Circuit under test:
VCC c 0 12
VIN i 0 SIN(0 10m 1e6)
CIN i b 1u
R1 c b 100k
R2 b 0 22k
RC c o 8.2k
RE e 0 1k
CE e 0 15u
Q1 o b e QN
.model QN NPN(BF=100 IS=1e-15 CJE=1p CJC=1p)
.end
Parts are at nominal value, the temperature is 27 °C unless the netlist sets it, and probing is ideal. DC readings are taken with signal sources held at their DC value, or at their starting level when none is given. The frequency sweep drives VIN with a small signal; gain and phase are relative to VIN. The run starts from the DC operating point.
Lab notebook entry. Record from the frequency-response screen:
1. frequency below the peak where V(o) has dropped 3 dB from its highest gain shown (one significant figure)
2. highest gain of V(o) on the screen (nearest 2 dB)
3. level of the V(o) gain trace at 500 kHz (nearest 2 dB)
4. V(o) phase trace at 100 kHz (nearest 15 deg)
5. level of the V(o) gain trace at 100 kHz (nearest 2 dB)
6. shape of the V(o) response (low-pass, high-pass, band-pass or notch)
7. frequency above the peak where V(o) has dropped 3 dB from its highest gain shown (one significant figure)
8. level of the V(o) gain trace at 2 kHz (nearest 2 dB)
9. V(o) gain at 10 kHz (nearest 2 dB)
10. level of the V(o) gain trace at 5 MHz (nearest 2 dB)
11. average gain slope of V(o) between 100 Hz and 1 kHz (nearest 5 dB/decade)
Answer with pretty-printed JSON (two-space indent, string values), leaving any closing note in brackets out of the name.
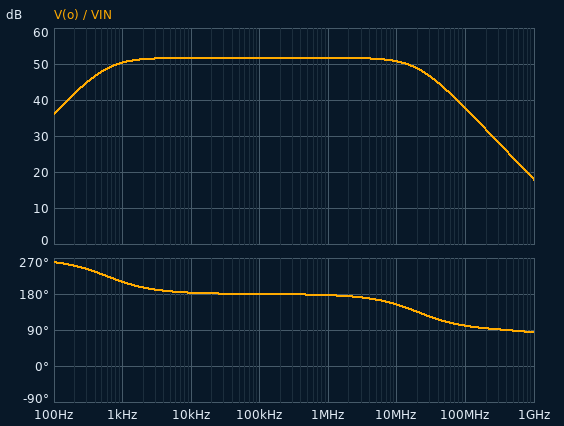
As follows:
{
  "frequency below the peak where V(o) has dropped 3 dB from its highest gain shown": "600 Hz",
  "highest gain of V(o) on the screen": "52 dB",
  "level of the V(o) gain trace at 500 kHz": "52 dB",
  "V(o) phase trace at 100 kHz": "180 deg",
  "level of the V(o) gain trace at 100 kHz": "52 dB",
  "shape of the V(o) response": "band-pass",
  "frequency above the peak where V(o) has dropped 3 dB from its highest gain shown": "20 MHz",
  "level of the V(o) gain trace at 2 kHz": "52 dB",
  "V(o) gain at 10 kHz": "52 dB",
  "level of the V(o) gain trace at 5 MHz": "52 dB",
  "average gain slope of V(o) between 100 Hz and 1 kHz": "15 dB/decade"
}
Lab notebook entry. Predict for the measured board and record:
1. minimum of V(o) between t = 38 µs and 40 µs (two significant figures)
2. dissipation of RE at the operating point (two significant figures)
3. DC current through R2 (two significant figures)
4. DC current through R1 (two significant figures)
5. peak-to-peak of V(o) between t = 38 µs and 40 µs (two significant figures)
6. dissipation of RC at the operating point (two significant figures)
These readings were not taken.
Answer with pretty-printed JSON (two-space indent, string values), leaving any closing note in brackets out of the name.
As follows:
{
  "minimum of V(o) between t = 38 µs and 40 µs": "1.3 V",
  "dissipation of RE at the operating point": "1.5 mW",
  "DC current through R2": "88 µA",
  "DC current through R1": "100 µA",
  "peak-to-peak of V(o) between t = 38 µs and 40 µs": "4.4 V",
  "dissipation of RC at the operating point": "12 mW"
}
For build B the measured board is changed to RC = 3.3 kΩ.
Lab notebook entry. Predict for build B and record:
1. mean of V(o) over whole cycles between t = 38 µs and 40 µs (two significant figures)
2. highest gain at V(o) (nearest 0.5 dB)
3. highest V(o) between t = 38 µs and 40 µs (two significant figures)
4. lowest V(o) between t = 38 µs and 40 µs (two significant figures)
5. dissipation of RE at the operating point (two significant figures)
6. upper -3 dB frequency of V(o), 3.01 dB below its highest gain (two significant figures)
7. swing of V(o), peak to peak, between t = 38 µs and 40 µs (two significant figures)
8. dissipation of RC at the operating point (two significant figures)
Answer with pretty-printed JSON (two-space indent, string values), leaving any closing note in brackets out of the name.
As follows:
{
  "mean of V(o) over whole cycles between t = 38 µs and 40 µs": "7.9 V",
  "highest gain at V(o)": "44.0 dB",
  "highest V(o) between t = 38 µs and 40 µs": "9.3 V",
  "lowest V(o) between t = 38 µs and 40 µs": "6.1 V",
  "dissipation of RE at the operating point": "1.5 mW",
  "upper -3 dB frequency of V(o), 3.01 dB below its highest gain": "100 MHz",
  "swing of V(o), peak to peak, between t = 38 µs and 40 µs": "3.2 V",
  "dissipation of RC at the operating point": "4.9 mW"
}
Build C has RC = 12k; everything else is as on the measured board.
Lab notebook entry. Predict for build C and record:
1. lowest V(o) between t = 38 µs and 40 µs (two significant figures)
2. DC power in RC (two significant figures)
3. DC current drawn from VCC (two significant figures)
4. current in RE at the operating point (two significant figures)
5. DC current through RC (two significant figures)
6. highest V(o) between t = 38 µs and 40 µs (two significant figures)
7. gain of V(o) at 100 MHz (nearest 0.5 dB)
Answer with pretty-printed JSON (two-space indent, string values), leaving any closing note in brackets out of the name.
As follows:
{
  "lowest V(o) between t = 38 µs and 40 µs": "990 mV",
  "DC power in RC": "10 mW",
  "DC current drawn from VCC": "1.0 mA",
  "current in RE at the operating point": "940 µA",
  "DC current through RC": "910 µA",
  "highest V(o) between t = 38 µs and 40 µs": "4.8 V",
  "gain of V(o) at 100 MHz": "26.0 dB"
}
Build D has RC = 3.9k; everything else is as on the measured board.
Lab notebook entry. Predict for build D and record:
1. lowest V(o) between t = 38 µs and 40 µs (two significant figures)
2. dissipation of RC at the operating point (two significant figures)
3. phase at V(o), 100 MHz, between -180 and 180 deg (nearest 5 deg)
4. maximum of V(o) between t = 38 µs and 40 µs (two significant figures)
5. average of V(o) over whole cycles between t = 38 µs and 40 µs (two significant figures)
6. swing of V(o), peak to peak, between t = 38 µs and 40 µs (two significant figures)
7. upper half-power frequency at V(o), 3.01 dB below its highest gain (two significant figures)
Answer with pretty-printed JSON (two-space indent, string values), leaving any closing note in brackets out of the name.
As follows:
{
  "lowest V(o) between t = 38 µs and 40 µs": "5.1 V",
  "dissipation of RC at the operating point": "5.7 mW",
  "phase at V(o), 100 MHz, between -180 and 180 deg": "130 deg",
  "maximum of V(o) between t = 38 µs and 40 µs": "8.8 V",
  "average of V(o) over whole cycles between t = 38 µs and 40 µs": "7.1 V",
  "swing of V(o), peak to peak, between t = 38 µs and 40 µs": "3.7 V",
  "upper half-power frequency at V(o), 3.01 dB below its highest gain": "81 MHz"
}
